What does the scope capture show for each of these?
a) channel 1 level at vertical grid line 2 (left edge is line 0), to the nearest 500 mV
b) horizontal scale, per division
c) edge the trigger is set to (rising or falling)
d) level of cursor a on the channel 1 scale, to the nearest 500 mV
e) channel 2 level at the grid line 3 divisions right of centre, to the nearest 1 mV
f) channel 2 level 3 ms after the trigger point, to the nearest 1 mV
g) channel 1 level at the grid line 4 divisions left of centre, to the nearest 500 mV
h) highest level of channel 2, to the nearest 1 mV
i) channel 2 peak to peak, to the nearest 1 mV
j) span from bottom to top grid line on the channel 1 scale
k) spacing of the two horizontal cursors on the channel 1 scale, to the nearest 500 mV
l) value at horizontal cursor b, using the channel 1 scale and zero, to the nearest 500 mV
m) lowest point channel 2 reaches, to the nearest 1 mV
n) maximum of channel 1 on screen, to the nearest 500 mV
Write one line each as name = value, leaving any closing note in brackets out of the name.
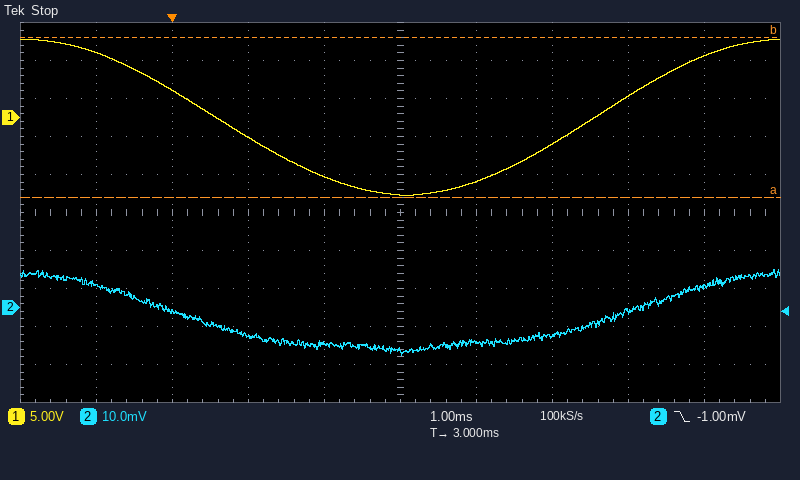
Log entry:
channel 1 level at vertical grid line 2 (left edge is line 0), to the nearest 500 mV = 3.5 V
horizontal scale, per division = 1 ms
edge the trigger is set to = falling
level of cursor a on the channel 1 scale, to the nearest 500 mV = -10.5 V
channel 2 level at the grid line 3 divisions right of centre, to the nearest 1 mV = -1 mV
channel 2 level 3 ms after the trigger point, to the nearest 1 mV = -12 mV
channel 1 level at the grid line 4 divisions left of centre, to the nearest 500 mV = 8.5 V
highest level of channel 2, to the nearest 1 mV = 10 mV
channel 2 peak to peak, to the nearest 1 mV = 23 mV
span from bottom to top grid line on the channel 1 scale = 50 V
spacing of the two horizontal cursors on the channel 1 scale, to the nearest 500 mV = 21.0 V
value at horizontal cursor b, using the channel 1 scale and zero, to the nearest 500 mV = 10.5 V
lowest point channel 2 reaches, to the nearest 1 mV = -13 mV
maximum of channel 1 on screen, to the nearest 500 mV = 10.5 V
